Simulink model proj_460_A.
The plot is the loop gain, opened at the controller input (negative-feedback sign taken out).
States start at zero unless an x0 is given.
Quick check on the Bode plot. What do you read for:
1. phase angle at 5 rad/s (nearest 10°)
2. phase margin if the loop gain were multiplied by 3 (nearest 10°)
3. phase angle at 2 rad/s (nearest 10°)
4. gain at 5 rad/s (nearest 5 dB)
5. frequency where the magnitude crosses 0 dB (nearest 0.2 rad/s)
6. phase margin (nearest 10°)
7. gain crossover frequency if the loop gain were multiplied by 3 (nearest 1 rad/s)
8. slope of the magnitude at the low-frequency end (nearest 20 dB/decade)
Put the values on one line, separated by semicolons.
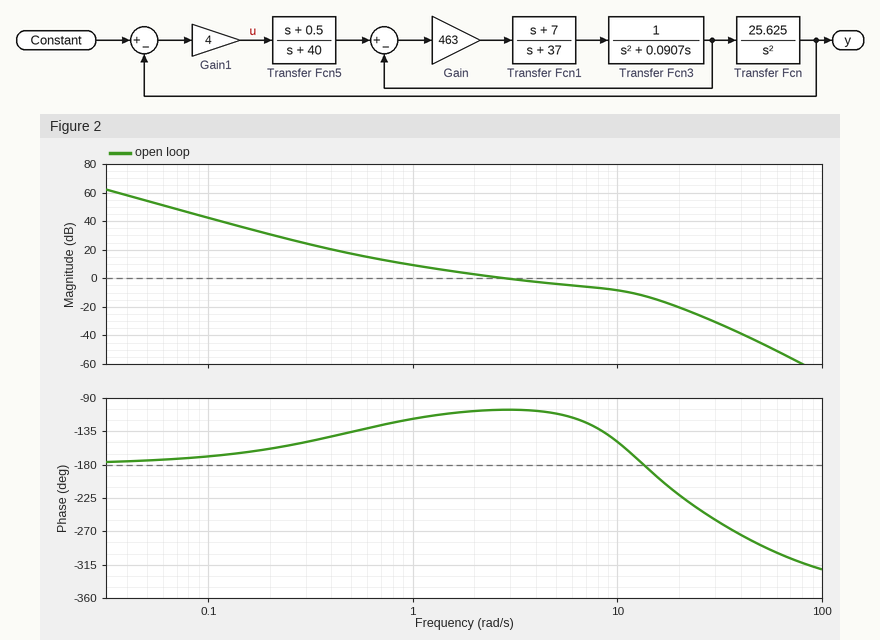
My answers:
-110°; 20°; -110°; -5 dB; 2.8 rad/s; 70°; 11 rad/s; -40 dB/decade
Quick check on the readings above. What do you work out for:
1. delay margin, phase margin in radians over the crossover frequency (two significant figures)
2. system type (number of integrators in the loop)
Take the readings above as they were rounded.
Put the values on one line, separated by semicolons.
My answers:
0.44 s; 2
